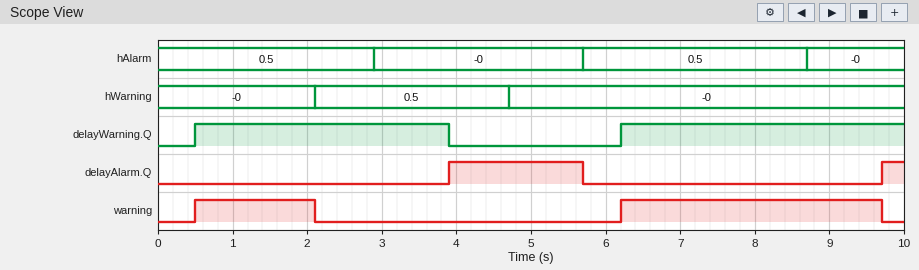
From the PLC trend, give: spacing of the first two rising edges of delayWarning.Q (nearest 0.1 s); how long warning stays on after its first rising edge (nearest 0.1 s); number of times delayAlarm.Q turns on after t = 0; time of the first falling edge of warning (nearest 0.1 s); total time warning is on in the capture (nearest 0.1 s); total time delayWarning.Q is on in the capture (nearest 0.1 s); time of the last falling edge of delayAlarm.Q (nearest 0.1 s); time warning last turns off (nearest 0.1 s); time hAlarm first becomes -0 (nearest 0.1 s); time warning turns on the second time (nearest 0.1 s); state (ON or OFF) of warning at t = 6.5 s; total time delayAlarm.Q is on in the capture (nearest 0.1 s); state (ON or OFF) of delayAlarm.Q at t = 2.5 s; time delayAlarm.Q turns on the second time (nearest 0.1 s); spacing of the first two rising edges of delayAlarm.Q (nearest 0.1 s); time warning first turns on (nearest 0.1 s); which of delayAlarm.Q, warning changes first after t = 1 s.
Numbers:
5.7 s
1.6 s
2
2.1 s
5.1 s
7.2 s
5.7 s
9.7 s
2.9 s
6.2 s
ON
2.1 s
OFF
9.7 s
5.8 s
0.5 s
warning
